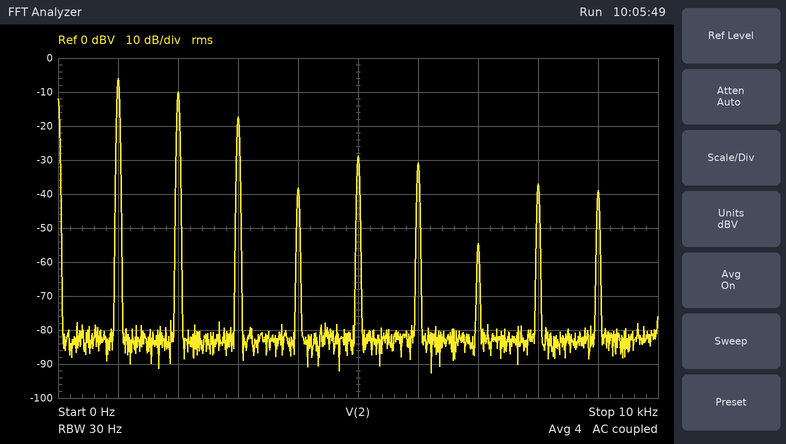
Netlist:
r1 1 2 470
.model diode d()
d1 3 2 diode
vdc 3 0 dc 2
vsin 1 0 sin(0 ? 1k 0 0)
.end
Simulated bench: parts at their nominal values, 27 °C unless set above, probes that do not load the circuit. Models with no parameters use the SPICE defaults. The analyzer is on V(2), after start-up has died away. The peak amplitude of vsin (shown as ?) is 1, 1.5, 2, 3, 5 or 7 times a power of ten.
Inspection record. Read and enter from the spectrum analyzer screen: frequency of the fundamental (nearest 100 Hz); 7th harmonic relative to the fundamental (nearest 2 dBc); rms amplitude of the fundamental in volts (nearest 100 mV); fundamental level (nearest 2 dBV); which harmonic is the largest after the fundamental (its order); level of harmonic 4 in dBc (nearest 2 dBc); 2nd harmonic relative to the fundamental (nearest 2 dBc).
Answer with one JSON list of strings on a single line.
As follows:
["1.0 kHz", "-48 dBc", "500 mV", "-6 dBV", "2", "-32 dBc", "-4 dBc"]
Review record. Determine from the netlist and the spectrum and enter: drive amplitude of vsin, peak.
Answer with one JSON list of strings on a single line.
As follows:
["3 V"]
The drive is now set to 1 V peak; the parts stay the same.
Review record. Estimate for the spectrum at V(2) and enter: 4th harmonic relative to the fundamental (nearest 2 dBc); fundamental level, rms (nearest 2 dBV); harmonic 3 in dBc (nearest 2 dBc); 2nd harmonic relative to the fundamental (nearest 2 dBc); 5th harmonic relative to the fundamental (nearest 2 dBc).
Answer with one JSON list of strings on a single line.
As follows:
["-34 dBc", "-36 dBV", "-24 dBc", "-14 dBc", "-44 dBc"]
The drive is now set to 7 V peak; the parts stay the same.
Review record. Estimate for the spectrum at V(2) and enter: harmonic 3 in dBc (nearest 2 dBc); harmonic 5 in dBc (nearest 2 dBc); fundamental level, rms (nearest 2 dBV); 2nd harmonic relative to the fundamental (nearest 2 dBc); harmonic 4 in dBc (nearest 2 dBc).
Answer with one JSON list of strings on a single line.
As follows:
["-20 dBc", "-26 dBc", "6 dBV", "-6 dBc", "-22 dBc"]
